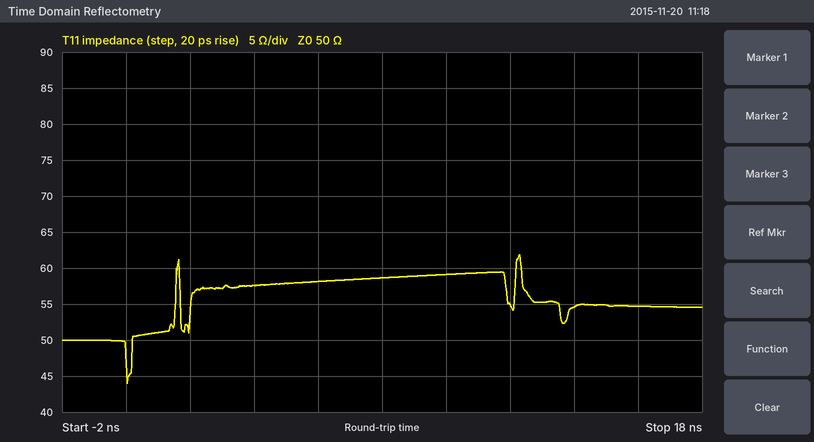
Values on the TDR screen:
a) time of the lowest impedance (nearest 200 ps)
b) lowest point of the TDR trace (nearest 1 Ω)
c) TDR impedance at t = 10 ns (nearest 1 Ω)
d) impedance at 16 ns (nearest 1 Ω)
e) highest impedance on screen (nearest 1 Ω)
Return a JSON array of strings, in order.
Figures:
["0.0 ns", "44 Ω", "59 Ω", "55 Ω", "62 Ω"]
